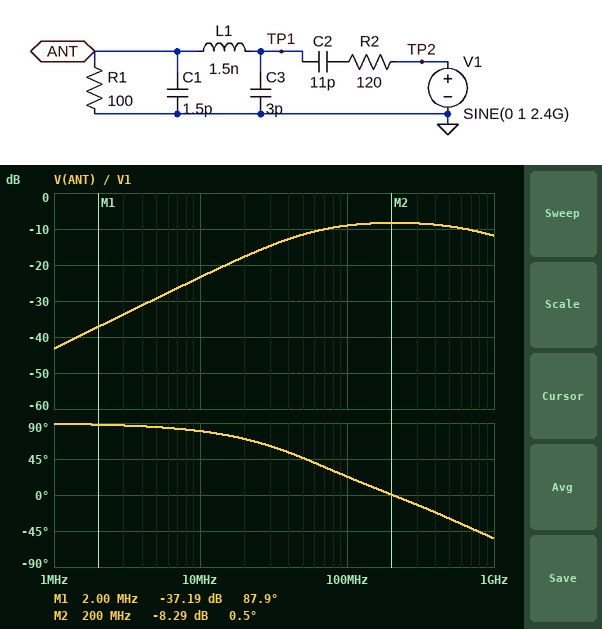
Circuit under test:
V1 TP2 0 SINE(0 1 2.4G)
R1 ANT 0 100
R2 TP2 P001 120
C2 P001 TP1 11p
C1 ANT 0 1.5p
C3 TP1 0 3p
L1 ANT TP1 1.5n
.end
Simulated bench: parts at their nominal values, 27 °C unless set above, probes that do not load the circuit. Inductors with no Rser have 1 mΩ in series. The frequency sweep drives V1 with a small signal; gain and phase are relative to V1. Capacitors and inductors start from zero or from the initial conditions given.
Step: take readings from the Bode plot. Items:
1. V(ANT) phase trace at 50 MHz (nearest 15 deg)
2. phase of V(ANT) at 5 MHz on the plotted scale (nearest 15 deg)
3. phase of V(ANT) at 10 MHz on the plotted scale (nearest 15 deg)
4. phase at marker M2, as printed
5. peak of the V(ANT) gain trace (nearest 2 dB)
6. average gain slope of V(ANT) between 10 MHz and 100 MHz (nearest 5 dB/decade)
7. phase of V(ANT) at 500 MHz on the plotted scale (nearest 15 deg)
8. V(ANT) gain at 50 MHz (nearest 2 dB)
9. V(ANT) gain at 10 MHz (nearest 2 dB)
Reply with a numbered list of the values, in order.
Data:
1. 45 deg
2. 90 deg
3. 75 deg
4. 0.5 deg
5. -8 dB
6. 15 dB/decade
7. -30 deg
8. -12 dB
9. -24 dB
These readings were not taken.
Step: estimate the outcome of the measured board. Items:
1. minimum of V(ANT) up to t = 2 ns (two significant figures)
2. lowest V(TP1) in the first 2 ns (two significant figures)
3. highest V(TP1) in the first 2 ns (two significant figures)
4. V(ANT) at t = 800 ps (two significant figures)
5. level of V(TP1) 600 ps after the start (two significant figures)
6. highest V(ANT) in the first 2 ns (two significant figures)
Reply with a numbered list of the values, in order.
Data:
1. -190 mV
2. -100 mV
3. 160 mV
4. -170 mV
5. 98 mV
6. 230 mV
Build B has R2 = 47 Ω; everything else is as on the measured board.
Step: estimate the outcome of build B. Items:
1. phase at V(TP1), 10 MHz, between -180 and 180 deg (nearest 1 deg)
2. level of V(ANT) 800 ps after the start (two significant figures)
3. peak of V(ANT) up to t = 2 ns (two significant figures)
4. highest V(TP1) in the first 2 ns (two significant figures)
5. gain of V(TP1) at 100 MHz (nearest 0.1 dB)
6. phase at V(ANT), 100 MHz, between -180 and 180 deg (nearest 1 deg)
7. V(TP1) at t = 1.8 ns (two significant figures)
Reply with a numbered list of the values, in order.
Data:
1. 83 deg
2. -410 mV
3. 450 mV
4. 320 mV
5. -7.2 dB
6. 35 deg
7. 200 mV
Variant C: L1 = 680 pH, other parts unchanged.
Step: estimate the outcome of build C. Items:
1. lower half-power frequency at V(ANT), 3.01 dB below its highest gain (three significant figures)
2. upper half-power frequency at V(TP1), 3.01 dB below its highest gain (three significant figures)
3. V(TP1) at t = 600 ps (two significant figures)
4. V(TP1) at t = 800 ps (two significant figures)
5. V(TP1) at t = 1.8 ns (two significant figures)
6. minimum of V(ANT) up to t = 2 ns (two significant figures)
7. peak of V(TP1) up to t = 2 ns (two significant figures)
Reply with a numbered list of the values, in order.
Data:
1. 52.1 MHz
2. 811 MHz
3. 110 mV
4. -110 mV
5. 73 mV
6. -150 mV
7. 150 mV
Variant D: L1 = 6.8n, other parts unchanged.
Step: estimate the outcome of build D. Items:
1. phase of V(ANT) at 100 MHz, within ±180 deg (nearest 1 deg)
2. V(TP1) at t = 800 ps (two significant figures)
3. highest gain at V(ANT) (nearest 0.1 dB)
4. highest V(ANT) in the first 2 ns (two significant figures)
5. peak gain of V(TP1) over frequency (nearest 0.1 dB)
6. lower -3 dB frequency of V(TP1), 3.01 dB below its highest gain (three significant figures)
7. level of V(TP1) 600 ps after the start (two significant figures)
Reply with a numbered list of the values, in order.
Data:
1. 22 deg
2. -270 mV
3. -8.1 dB
4. 190 mV
5. -8.2 dB
6. 52.4 MHz
7. 260 mV
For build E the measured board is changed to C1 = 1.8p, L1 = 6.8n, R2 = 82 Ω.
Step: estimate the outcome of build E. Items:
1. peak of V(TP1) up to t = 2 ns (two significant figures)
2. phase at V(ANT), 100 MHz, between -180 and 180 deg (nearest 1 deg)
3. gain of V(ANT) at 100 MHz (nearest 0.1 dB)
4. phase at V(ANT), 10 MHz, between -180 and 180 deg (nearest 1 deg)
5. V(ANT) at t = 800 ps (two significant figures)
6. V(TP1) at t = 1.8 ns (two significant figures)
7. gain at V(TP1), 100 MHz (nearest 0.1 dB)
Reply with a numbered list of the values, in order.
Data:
1. 370 mV
2. 27 deg
3. -8.0 dB
4. 81 deg
5. 180 mV
6. 270 mV
7. -8.1 dB
